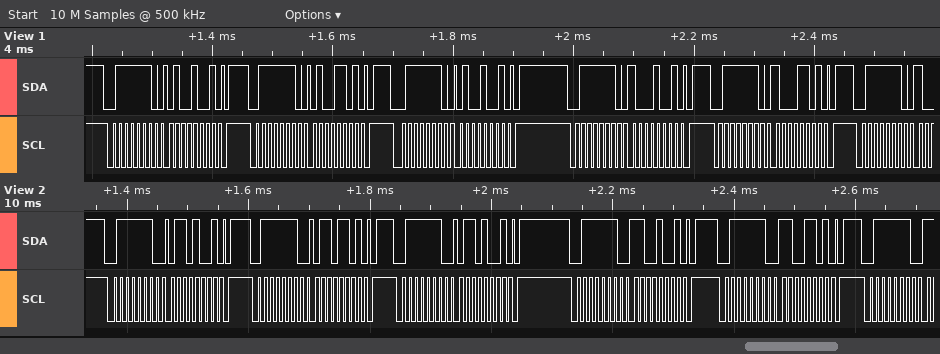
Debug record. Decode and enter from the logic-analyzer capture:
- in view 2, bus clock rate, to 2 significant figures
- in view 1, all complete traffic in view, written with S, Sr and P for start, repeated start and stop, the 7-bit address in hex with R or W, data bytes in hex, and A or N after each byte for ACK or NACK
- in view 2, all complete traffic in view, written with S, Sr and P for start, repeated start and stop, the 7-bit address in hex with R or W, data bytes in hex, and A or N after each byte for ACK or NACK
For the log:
100 kHz
S 3FW A 49 A P S 3FW A 4D A P S 3FW A 49 A P S 3FW A 89 A P S 3FW A 8D A P S 3FW A
S 3FW A 69 A P S 3FW A 6D A P S 3FW A 69 A P S 3FW A C9 A P S 3FW A CD A P S 3FW A
